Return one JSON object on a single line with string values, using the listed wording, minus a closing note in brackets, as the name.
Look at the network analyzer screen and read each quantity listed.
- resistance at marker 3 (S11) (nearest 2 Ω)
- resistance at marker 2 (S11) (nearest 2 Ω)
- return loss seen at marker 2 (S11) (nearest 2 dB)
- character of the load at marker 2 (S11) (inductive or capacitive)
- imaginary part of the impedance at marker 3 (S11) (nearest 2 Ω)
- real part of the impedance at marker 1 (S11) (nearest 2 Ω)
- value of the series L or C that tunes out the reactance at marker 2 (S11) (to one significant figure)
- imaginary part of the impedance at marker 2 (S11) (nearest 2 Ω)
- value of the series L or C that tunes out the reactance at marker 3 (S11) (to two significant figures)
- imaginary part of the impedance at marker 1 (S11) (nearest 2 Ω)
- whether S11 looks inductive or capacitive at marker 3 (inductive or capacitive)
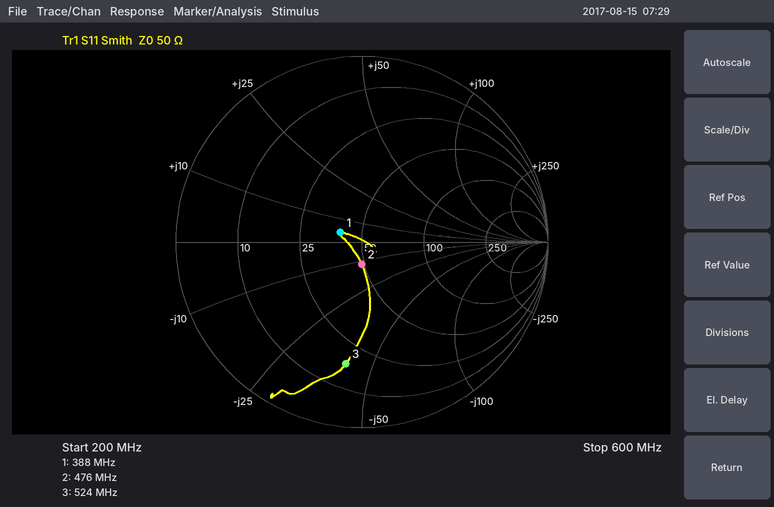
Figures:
{"resistance at marker 3 (S11)": "18 Ω", "resistance at marker 2 (S11)": "48 Ω", "return loss seen at marker 2 (S11)": "18 dB", "character of the load at marker 2 (S11)": "capacitive", "imaginary part of the impedance at marker 3 (S11)": "-40 Ω", "real part of the impedance at marker 1 (S11)": "40 Ω", "value of the series L or C that tunes out the reactance at marker 2 (S11)": "4 nH", "imaginary part of the impedance at marker 2 (S11)": "-12 Ω", "value of the series L or C that tunes out the reactance at marker 3 (S11)": "12 nH", "imaginary part of the impedance at marker 1 (S11)": "+4 Ω", "whether S11 looks inductive or capacitive at marker 3": "capacitive"}
